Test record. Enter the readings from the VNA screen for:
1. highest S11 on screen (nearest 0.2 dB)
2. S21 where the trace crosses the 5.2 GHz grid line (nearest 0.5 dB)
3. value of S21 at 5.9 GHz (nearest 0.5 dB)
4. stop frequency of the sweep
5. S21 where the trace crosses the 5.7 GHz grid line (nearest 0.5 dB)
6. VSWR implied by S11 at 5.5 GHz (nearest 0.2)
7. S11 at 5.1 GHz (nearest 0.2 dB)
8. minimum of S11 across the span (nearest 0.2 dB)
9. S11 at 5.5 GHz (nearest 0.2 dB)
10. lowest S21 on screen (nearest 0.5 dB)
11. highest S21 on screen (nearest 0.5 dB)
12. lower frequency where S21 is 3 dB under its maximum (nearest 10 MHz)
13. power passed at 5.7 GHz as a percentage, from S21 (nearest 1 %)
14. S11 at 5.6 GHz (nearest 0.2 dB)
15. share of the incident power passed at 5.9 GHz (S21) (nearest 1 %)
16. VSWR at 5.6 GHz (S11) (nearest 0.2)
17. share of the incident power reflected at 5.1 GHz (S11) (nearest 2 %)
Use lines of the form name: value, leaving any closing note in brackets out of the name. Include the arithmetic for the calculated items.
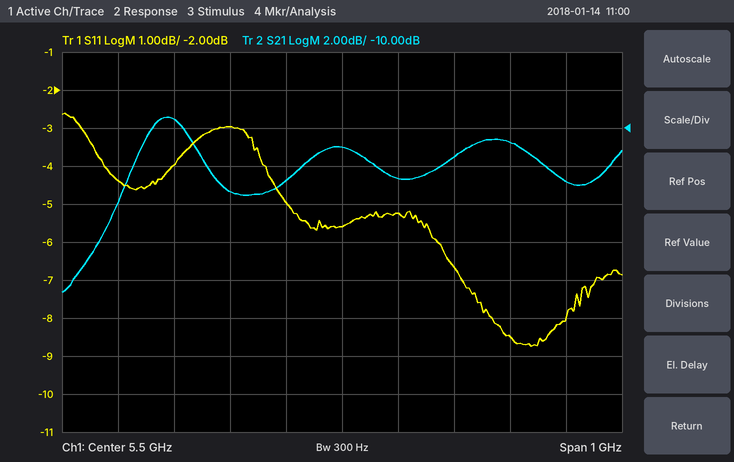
highest S11 on screen: -2.6 dB
S21 where the trace crosses the 5.2 GHz grid line: -9.5 dB
value of S21 at 5.9 GHz: -13.0 dB
stop frequency of the sweep: 6 GHz
S21 where the trace crosses the 5.7 GHz grid line: -11.5 dB
VSWR implied by S11 at 5.5 GHz: |Γ| = 10^(-5.6/20) = 0.5248; VSWR = (1 + 0.5248)/(1 − 0.5248) ≈ 3.2
S11 at 5.1 GHz: -4.4 dB
minimum of S11 across the span: -8.8 dB
S11 at 5.5 GHz: -5.6 dB
lowest S21 on screen: -18.5 dB
highest S21 on screen: -9.5 dB
lower frequency where S21 is 3 dB under its maximum: 5.12 GHz
power passed at 5.7 GHz as a percentage, from S21: 10^(-11.5/10) ≈ 7 %
S11 at 5.6 GHz: -5.2 dB
share of the incident power passed at 5.9 GHz (S21): 10^(-13/10) ≈ 5 %
VSWR at 5.6 GHz (S11): |Γ| = 10^(-5.2/20) = 0.5495; VSWR = (1 + 0.5495)/(1 − 0.5495) ≈ 3.4
share of the incident power reflected at 5.1 GHz (S11): 10^(-4.4/10) ≈ 36 %
